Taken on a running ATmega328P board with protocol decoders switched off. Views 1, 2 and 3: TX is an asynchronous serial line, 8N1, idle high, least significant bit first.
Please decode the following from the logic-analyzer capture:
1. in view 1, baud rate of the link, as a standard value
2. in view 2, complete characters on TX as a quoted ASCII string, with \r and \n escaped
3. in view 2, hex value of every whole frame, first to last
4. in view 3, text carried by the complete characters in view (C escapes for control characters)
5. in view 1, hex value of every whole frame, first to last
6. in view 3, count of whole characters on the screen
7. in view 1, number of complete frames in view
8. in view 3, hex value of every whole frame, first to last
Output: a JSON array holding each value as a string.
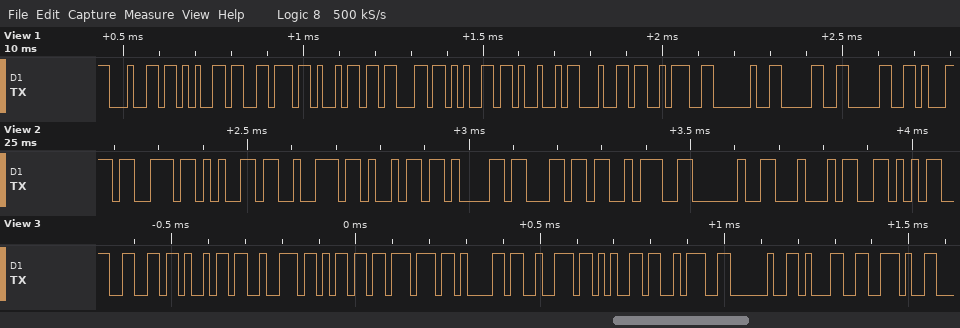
["57600 baud", "\"serial: DV\"", "0x73 0x65 0x72 0x69 0x61 0x6C 0x3A 0x20 0x44 0x56", "\"firmware: 1.\"", "64 65 76 69 63 65 49 64 3A 20 30 30", "12", "12", "66 69 72 6D 77 61 72 65 3A 20 31 2E"]
